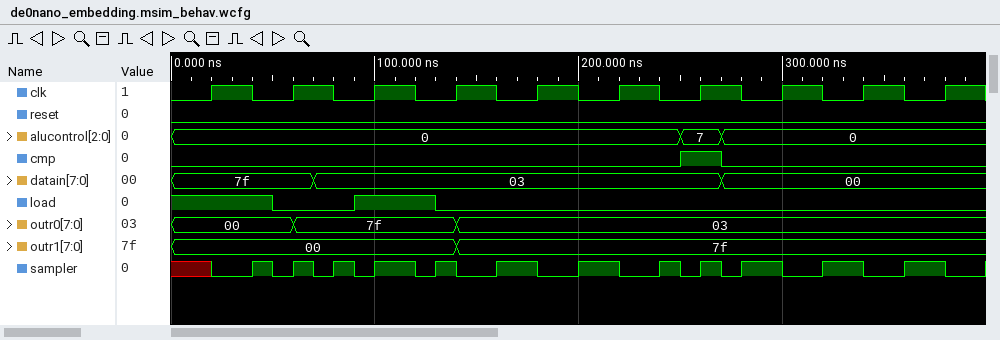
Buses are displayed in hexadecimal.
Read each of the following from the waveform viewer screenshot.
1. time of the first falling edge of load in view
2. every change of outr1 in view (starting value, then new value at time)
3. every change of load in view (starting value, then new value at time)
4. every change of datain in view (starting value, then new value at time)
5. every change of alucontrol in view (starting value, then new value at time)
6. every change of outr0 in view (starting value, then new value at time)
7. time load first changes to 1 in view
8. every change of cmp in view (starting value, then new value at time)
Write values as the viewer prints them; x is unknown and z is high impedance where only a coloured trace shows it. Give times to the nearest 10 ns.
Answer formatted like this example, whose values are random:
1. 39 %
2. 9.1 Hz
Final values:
1. 50 ns
2. 00, 7f at 140 ns
3. 1, 0 at 50 ns, 1 at 90 ns, 0 at 130 ns
4. 7f, 03 at 70 ns, 00 at 270 ns
5. 0, 7 at 250 ns, 0 at 270 ns
6. 00, 7f at 60 ns, 03 at 140 ns
7. 90 ns
8. 0, 1 at 250 ns, 0 at 270 ns
